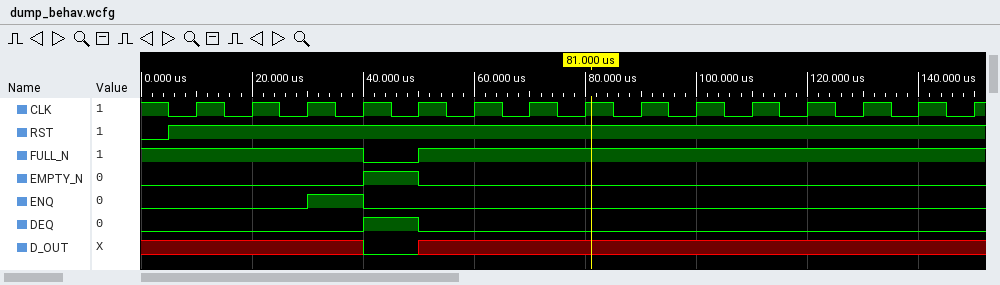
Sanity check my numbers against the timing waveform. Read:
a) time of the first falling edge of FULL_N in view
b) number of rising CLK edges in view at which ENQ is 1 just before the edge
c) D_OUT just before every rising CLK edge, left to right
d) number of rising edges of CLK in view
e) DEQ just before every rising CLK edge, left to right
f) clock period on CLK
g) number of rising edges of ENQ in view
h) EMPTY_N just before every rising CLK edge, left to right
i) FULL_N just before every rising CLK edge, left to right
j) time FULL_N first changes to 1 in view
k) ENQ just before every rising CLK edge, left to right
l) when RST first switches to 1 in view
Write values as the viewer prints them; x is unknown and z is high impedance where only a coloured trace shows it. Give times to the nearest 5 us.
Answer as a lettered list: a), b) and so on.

a) 40 us
b) 1
c) x x x x 0 x x x x x x x x x x
d) 15
e) 0 0 0 0 1 0 0 0 0 0 0 0 0 0 0
f) 10 us
g) 1
h) 0 0 0 0 1 0 0 0 0 0 0 0 0 0 0
i) 1 1 1 1 0 1 1 1 1 1 1 1 1 1 1
j) 50 us
k) 0 0 0 1 0 0 0 0 0 0 0 0 0 0 0
l) 5 us
